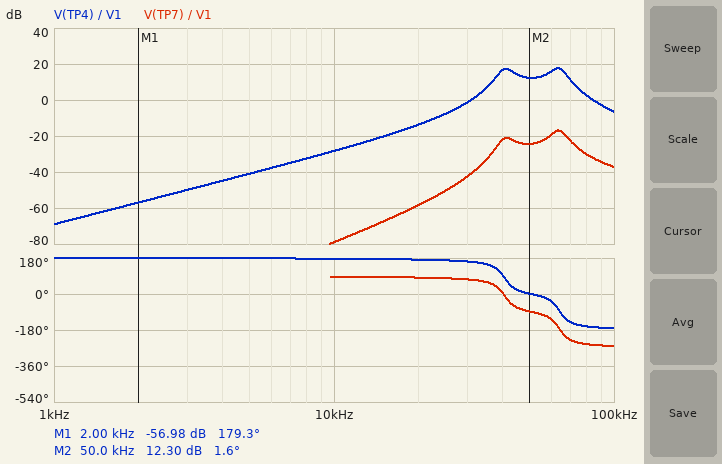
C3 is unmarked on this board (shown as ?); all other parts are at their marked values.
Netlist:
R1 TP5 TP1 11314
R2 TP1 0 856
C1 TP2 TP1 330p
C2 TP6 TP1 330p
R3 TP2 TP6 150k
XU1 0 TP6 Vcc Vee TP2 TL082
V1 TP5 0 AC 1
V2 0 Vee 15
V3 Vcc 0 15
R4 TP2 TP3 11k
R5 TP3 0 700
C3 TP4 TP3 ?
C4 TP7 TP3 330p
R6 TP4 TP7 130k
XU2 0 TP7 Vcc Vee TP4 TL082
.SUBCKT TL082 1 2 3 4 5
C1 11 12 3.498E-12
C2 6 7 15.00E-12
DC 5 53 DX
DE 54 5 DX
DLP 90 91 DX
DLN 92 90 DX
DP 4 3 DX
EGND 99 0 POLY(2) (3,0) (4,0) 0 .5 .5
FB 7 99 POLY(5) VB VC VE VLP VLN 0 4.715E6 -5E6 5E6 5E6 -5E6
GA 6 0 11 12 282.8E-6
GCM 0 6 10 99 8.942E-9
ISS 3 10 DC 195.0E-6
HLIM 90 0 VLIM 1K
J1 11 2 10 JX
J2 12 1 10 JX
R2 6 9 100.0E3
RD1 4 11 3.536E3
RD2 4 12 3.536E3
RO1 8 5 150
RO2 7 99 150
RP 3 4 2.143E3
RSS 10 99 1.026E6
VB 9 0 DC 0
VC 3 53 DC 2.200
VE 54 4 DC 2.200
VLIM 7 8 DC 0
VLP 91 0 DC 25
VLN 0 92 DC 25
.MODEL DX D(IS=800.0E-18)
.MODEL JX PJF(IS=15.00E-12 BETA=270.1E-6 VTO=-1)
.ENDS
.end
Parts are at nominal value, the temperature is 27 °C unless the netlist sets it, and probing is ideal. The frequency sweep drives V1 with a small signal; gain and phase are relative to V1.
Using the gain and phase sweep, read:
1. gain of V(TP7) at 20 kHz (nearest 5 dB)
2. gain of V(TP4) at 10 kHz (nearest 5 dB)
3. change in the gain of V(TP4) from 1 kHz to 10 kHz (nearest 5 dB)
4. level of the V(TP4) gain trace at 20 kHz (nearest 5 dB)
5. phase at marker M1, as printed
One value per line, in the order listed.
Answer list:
-60 dB
-30 dB
40 dB
-15 dB
179.3 deg
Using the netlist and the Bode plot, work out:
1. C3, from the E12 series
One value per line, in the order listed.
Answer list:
150 pF
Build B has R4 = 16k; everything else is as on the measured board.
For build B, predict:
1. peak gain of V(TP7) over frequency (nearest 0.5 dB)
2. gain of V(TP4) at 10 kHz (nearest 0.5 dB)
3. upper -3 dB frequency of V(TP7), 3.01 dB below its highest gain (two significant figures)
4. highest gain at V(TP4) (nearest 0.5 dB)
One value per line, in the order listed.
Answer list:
-20.0 dB
-31.5 dB
67 kHz
14.5 dB
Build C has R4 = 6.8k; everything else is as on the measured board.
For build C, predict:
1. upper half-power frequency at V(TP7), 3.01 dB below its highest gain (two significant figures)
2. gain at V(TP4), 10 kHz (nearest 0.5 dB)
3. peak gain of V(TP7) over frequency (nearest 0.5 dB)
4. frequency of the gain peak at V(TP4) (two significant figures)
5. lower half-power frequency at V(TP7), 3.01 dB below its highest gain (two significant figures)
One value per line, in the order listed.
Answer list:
68 kHz
-24.5 dB
-13.0 dB
64 kHz
60 kHz
